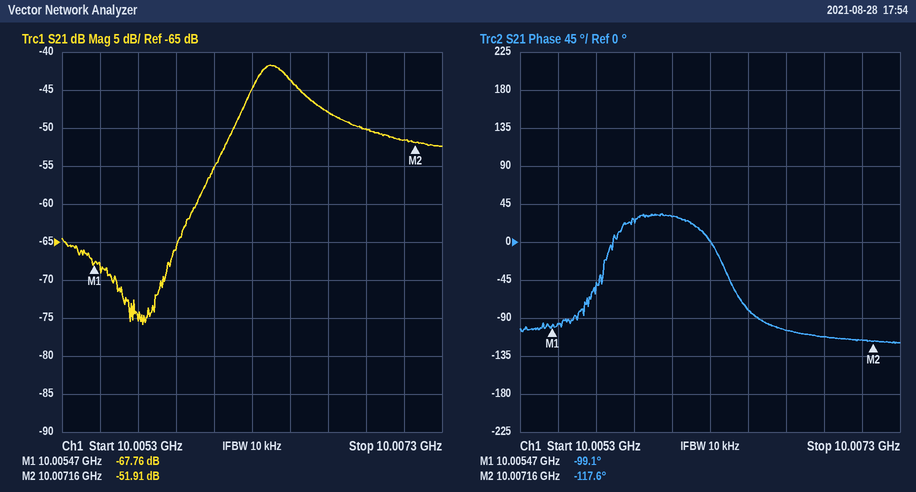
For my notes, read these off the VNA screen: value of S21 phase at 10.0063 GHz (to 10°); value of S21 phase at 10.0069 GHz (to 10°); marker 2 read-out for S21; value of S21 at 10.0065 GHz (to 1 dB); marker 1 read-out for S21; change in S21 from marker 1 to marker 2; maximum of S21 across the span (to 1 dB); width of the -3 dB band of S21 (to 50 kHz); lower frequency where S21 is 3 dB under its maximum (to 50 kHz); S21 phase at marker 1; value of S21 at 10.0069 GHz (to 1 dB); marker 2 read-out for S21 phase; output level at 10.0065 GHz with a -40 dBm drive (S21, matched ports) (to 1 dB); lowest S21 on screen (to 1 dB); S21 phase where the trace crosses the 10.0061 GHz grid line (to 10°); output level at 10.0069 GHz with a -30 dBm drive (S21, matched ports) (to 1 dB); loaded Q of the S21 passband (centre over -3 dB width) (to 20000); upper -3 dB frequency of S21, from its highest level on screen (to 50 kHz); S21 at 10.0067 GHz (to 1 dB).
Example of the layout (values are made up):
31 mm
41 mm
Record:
0°
-110°
-51.91 dB
-44 dB
-67.76 dB
15.85 dB
-42 dB
250 kHz
10.00630 GHz
-99.1°
-50 dB
-117.6°
-84 dBm
-76 dB
30°
-80 dBm
40000
10.00655 GHz
-48 dB
